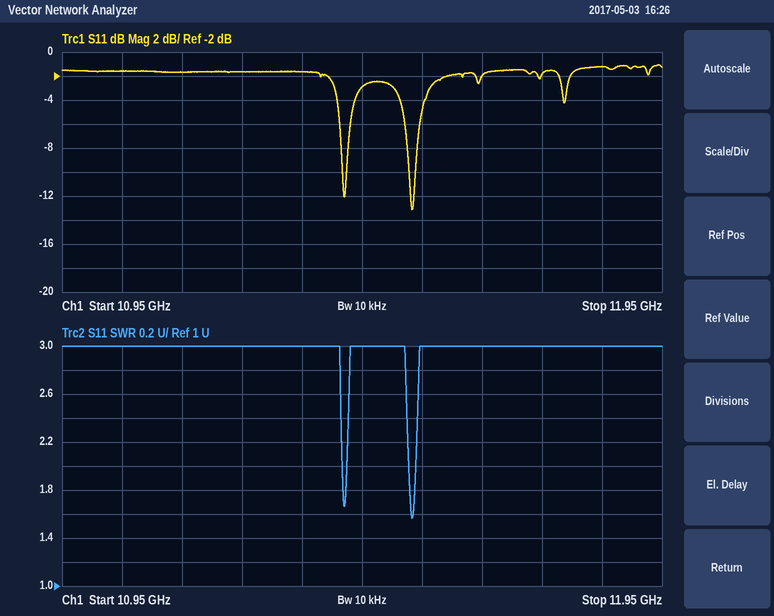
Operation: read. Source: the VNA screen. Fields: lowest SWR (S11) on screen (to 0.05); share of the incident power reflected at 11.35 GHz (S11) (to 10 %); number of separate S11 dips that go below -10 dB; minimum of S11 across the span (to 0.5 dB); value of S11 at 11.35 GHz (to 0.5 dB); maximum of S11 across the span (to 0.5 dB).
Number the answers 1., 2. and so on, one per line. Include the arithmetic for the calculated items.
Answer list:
1. 1.55
2. 10^(-1.5/10) ≈ 70.8 %, so 70 % to the nearest 10 %
3. 2
4. -13.0 dB
5. -1.5 dB
6. -1.0 dB
